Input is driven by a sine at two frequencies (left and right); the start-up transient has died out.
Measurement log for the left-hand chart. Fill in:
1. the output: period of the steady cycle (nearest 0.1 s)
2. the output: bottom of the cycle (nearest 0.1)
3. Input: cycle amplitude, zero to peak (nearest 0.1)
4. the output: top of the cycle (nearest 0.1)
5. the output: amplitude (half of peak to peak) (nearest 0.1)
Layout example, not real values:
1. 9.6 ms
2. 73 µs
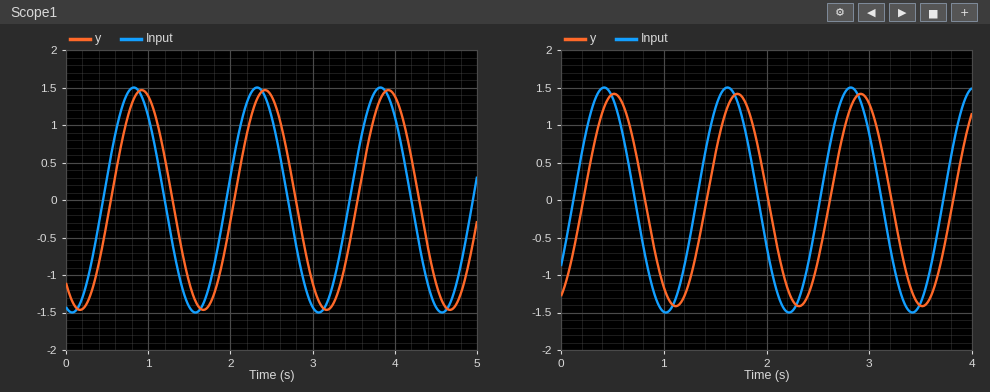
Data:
1. 1.5 s
2. -1.5
3. 1.5
4. 1.5
5. 1.5
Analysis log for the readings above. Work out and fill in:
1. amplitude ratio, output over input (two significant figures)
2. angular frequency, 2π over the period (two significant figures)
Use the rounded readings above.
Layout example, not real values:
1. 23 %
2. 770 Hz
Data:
1. 1.0
2. 4.2 rad/s
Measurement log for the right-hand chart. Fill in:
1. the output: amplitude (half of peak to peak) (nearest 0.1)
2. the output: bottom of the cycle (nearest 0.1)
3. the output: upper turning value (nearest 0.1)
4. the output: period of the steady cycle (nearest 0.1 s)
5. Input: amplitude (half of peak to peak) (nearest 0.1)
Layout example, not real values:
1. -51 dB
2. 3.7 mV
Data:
1. 1.4
2. -1.4
3. 1.4
4. 1.2 s
5. 1.5
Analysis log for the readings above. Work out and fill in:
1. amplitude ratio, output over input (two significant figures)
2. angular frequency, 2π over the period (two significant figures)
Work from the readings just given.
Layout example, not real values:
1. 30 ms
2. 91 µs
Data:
1. 0.93
2. 5.2 rad/s
